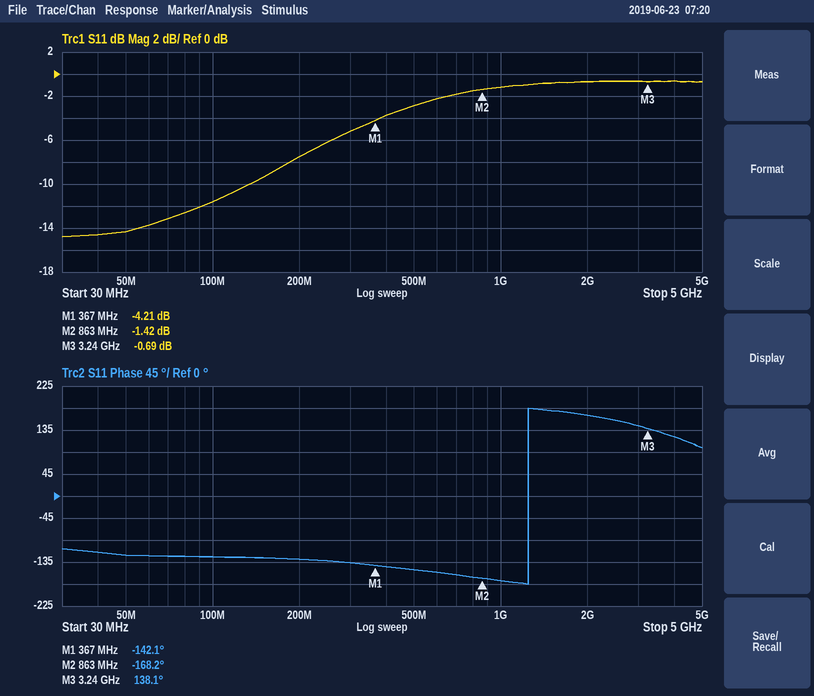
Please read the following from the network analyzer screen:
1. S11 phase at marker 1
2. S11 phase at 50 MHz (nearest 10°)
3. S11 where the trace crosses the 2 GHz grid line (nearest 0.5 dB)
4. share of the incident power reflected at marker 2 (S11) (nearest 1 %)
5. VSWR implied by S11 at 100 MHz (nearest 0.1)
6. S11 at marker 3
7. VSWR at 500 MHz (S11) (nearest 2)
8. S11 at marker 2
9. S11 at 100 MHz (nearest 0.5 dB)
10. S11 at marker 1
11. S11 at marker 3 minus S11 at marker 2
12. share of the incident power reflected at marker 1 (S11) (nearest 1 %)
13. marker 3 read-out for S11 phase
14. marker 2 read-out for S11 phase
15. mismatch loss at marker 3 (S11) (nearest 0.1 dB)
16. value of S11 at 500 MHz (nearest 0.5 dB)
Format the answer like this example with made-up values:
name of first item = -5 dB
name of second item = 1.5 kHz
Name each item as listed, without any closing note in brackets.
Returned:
S11 phase at marker 1 = -142.1°
S11 phase at 50 MHz = -120°
S11 where the trace crosses the 2 GHz grid line = -0.5 dB
share of the incident power reflected at marker 2 (S11) = 72 %
VSWR implied by S11 at 100 MHz = 1.7
S11 at marker 3 = -0.69 dB
VSWR at 500 MHz (S11) = 6
S11 at marker 2 = -1.42 dB
S11 at 100 MHz = -11.5 dB
S11 at marker 1 = -4.21 dB
S11 at marker 3 minus S11 at marker 2 = 0.73 dB
share of the incident power reflected at marker 1 (S11) = 38 %
marker 3 read-out for S11 phase = 138.1°
marker 2 read-out for S11 phase = -168.2°
mismatch loss at marker 3 (S11) = 8.3 dB
value of S11 at 500 MHz = -3.0 dB
